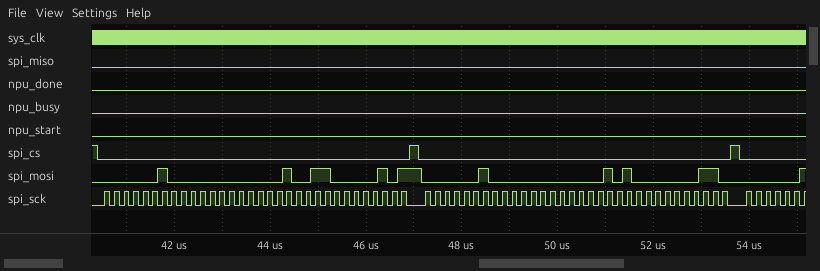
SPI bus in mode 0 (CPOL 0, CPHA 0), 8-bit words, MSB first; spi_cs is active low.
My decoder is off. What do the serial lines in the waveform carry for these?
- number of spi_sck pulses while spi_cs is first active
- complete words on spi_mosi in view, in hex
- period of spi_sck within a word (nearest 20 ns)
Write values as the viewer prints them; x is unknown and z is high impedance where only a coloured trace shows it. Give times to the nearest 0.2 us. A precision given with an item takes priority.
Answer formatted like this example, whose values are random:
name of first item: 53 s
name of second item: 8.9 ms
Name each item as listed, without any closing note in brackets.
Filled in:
number of spi_sck pulses while spi_cs is first active: 32
complete words on spi_mosi in view, in hex: 02, 00, 13, 05, 02, 00, 14, 06
period of spi_sck within a word: 200 ns
